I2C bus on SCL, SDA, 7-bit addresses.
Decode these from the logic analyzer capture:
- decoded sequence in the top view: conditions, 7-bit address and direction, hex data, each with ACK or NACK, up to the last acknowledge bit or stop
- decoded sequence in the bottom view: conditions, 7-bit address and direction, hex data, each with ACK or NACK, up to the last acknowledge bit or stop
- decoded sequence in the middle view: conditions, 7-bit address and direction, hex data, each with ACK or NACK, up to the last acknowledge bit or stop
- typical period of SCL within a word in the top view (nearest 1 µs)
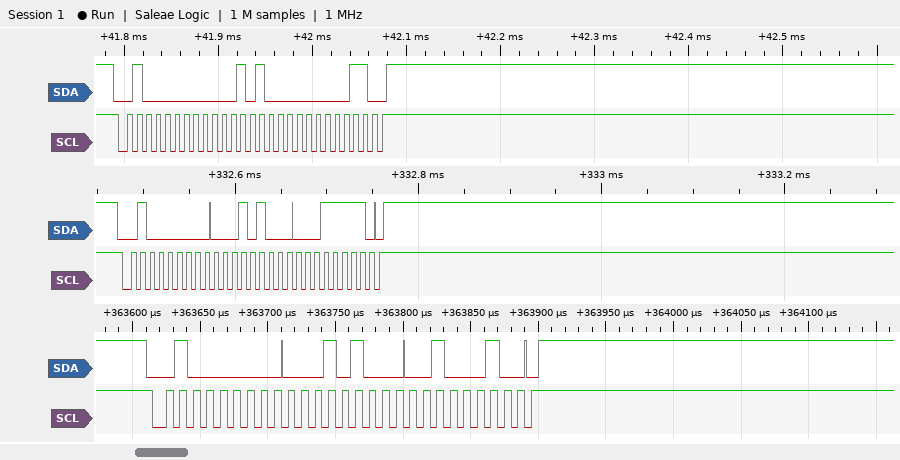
start, address 20 write ACK, 14 ACK, 03 ACK, stop
start, address 20 write ACK, 14 ACK, 22 ACK, stop
start, address 20 write ACK, 14 ACK, 1F ACK, stop
10 µs
